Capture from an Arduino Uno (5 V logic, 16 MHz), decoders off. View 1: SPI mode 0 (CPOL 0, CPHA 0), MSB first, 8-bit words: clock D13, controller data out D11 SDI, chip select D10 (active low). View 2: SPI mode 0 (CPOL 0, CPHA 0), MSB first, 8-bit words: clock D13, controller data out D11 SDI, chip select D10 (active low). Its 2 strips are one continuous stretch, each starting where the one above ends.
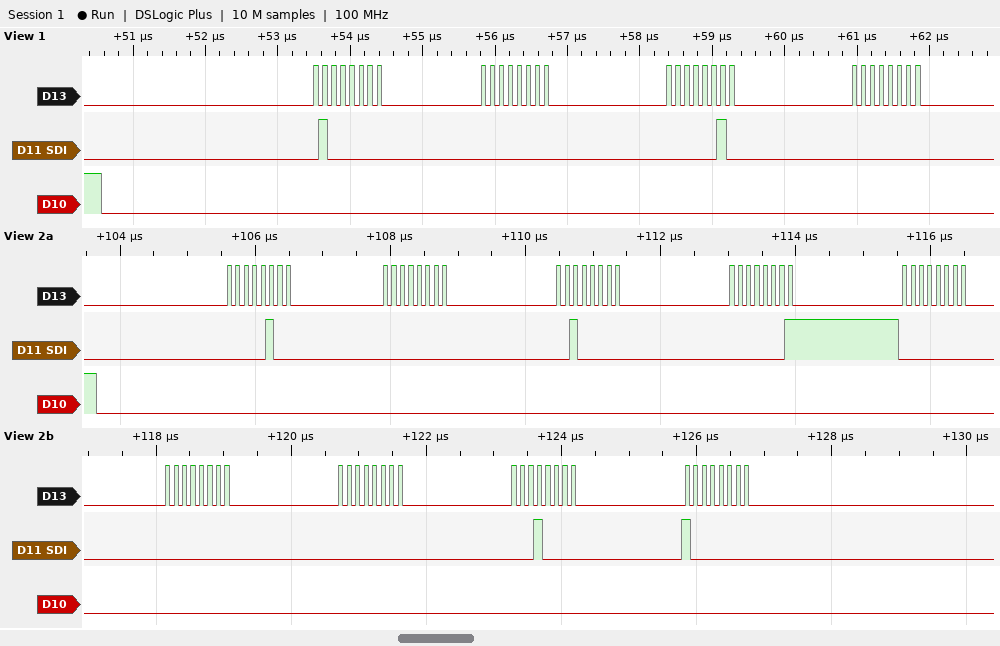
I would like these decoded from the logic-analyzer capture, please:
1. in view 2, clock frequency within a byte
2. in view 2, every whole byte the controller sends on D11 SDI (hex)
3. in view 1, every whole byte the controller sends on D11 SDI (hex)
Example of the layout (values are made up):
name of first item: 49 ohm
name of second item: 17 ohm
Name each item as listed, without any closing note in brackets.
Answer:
in view 2, clock frequency within a byte: 8 MHz
in view 2, every whole byte the controller sends on D11 SDI: 04 00 20 01 00 00 00 10 80
in view 1, every whole byte the controller sends on D11 SDI: 0x40 0x00 0x02 0x00
